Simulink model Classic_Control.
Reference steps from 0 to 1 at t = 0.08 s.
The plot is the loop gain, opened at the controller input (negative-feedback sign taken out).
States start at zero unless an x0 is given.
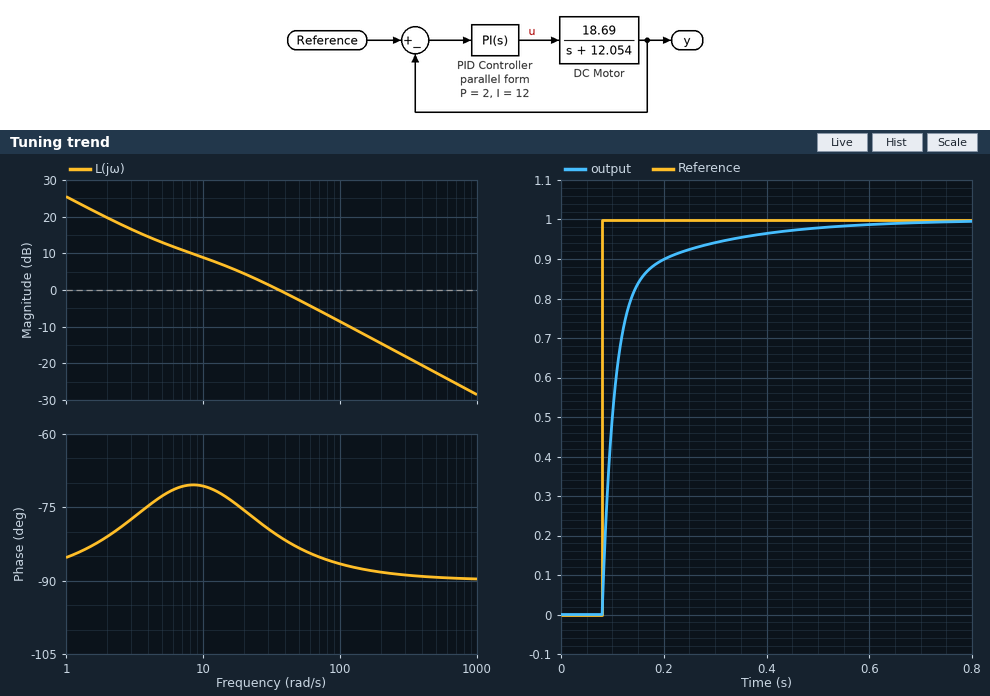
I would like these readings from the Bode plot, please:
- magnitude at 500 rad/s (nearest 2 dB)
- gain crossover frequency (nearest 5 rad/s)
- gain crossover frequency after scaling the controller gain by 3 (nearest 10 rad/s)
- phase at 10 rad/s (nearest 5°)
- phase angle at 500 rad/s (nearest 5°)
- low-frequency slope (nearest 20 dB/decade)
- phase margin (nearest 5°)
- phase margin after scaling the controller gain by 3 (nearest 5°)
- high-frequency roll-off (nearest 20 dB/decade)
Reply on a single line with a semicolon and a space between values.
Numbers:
-22 dB; 35 rad/s; 110 rad/s; -70°; -90°; -20 dB/decade; 100°; 95°; -20 dB/decade
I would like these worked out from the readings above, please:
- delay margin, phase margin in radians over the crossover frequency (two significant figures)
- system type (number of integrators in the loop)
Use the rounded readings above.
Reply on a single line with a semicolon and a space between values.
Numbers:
0.050 s; 1
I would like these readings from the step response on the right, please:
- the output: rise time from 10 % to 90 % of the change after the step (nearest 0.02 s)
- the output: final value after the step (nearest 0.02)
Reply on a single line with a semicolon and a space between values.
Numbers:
0.12 s; 1.00
